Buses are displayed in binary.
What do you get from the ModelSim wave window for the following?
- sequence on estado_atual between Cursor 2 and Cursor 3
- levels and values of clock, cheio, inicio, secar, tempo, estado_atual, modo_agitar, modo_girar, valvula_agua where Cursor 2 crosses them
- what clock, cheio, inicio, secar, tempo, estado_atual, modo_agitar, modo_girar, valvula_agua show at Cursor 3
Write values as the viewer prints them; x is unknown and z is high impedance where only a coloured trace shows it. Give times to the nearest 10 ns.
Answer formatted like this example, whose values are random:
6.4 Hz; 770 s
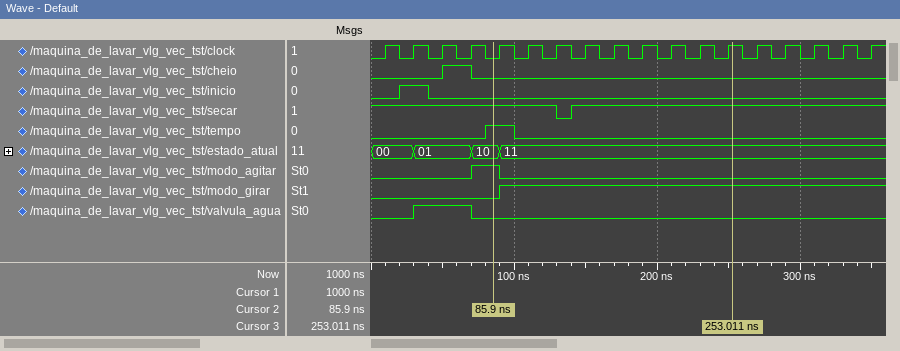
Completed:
10, 11; clock=0, cheio=0, inicio=0, secar=1, tempo=1, estado_atual=10, modo_agitar=1, modo_girar=0, valvula_agua=0; clock=1, cheio=0, inicio=0, secar=1, tempo=0, estado_atual=11, modo_agitar=0, modo_girar=1, valvula_agua=0
